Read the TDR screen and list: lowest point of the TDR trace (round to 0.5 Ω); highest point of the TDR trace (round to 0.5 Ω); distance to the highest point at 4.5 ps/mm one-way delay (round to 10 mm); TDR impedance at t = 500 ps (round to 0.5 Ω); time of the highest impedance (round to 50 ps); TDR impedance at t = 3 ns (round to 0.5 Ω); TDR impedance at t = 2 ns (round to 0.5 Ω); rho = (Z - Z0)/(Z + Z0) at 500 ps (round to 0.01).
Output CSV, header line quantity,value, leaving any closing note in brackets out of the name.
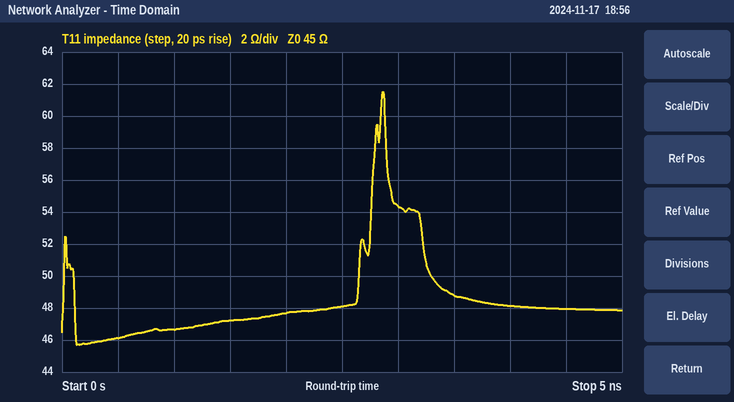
quantity,value
lowest point of the TDR trace,45.5 Ω
highest point of the TDR trace,61.5 Ω
distance to the highest point at 4.5 ps/mm one-way delay,320 mm
TDR impedance at t = 500 ps,46.0 Ω
time of the highest impedance,2.85 ns
TDR impedance at t = 3 ns,54.5 Ω
TDR impedance at t = 2 ns,47.5 Ω
rho = (Z - Z0)/(Z + Z0) at 500 ps,+0.01
